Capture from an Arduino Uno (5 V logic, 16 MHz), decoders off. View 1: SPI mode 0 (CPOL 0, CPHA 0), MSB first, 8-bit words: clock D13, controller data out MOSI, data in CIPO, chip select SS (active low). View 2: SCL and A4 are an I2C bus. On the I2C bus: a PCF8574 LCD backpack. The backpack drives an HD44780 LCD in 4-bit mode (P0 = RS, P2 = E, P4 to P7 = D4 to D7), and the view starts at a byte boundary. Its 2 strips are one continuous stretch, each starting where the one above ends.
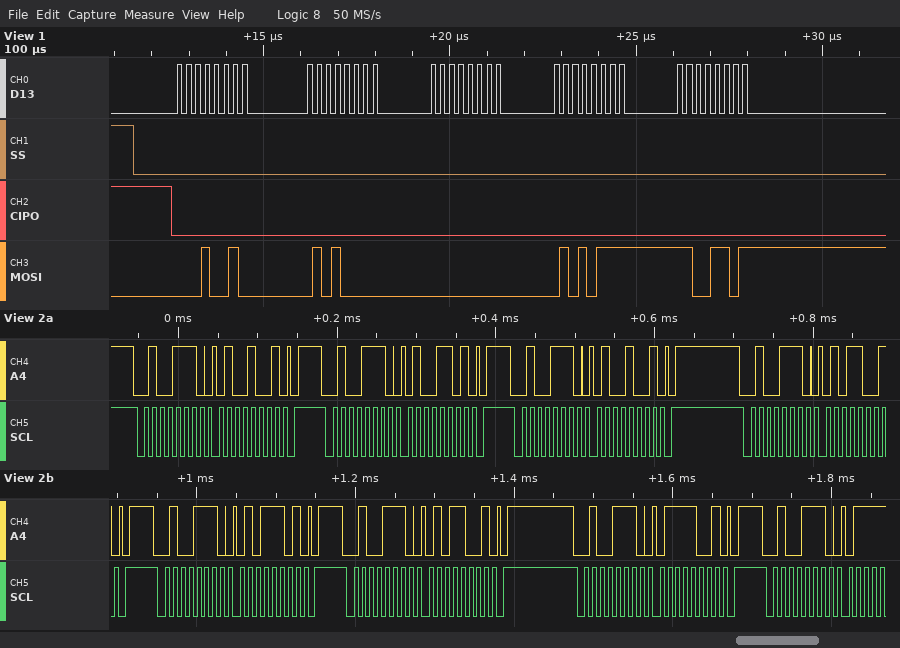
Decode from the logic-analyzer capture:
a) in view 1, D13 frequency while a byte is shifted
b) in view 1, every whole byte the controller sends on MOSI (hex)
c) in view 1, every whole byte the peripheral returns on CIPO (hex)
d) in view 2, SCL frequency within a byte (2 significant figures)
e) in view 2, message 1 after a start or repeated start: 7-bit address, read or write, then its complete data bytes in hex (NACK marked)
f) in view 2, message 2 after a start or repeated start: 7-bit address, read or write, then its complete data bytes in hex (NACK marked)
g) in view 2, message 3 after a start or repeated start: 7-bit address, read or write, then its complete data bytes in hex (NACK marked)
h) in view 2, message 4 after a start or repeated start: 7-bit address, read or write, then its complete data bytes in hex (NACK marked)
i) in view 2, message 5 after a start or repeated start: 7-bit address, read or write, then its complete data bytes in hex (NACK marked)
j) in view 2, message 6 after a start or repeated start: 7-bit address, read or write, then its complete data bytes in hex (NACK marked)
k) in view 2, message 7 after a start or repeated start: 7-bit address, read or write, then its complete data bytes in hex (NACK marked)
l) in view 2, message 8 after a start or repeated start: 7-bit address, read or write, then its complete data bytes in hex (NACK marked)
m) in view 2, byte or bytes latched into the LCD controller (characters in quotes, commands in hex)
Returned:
4 MHz
12 50 00 57 CD
00 00 00 00 00
100 kHz
0x27 write: 49
0x27 write: 4D
0x27 write: 49
0x27 write: 59
0x27 write: 5D
0x27 write: 59
0x27 write: 79
0x27 write
'E'
